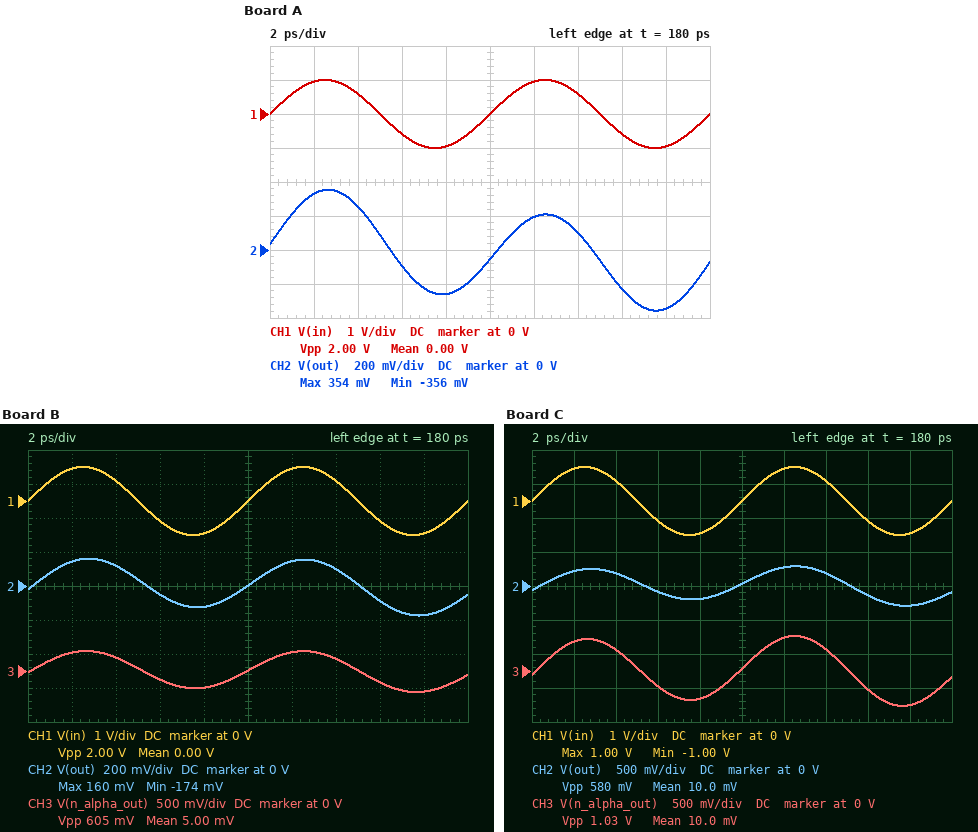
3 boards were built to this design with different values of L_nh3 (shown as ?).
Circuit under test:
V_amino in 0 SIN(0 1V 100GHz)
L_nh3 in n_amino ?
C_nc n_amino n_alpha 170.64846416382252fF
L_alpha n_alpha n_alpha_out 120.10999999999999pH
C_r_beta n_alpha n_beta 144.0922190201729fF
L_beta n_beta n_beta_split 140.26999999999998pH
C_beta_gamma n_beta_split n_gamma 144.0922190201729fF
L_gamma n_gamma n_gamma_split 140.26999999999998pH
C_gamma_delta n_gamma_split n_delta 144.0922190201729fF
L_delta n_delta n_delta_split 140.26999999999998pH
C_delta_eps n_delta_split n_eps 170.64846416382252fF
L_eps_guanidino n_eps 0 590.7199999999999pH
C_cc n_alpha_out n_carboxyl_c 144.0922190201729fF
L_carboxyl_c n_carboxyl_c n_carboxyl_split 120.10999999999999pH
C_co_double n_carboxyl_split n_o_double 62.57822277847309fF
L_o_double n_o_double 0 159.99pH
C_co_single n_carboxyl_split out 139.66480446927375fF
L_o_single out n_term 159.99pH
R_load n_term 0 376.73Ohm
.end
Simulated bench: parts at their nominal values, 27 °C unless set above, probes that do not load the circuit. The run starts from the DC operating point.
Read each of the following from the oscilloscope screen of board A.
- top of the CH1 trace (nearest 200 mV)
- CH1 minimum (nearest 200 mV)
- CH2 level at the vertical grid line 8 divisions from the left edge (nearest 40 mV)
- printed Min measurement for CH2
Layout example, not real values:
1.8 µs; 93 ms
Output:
1.0 V; -1.0 V; -240 mV; -356 mV
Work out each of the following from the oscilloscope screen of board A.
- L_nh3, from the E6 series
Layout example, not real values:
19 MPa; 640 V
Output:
68 pH
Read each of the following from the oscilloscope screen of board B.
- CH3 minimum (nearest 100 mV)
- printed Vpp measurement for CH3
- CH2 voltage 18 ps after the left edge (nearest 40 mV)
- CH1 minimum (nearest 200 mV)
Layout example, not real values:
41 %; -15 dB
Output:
-300 mV; 605 mV; -160 mV; -1.0 V
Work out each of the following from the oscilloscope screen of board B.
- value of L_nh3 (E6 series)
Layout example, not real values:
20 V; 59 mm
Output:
330 pH
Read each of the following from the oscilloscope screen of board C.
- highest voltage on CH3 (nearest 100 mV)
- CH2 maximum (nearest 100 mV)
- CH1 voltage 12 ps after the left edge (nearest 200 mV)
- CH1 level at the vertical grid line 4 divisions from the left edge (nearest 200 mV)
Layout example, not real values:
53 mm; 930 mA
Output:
500 mV; 300 mV; 1.0 V; -1.0 V
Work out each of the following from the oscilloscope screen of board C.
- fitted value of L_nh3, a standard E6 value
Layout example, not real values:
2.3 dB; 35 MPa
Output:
100 pH
